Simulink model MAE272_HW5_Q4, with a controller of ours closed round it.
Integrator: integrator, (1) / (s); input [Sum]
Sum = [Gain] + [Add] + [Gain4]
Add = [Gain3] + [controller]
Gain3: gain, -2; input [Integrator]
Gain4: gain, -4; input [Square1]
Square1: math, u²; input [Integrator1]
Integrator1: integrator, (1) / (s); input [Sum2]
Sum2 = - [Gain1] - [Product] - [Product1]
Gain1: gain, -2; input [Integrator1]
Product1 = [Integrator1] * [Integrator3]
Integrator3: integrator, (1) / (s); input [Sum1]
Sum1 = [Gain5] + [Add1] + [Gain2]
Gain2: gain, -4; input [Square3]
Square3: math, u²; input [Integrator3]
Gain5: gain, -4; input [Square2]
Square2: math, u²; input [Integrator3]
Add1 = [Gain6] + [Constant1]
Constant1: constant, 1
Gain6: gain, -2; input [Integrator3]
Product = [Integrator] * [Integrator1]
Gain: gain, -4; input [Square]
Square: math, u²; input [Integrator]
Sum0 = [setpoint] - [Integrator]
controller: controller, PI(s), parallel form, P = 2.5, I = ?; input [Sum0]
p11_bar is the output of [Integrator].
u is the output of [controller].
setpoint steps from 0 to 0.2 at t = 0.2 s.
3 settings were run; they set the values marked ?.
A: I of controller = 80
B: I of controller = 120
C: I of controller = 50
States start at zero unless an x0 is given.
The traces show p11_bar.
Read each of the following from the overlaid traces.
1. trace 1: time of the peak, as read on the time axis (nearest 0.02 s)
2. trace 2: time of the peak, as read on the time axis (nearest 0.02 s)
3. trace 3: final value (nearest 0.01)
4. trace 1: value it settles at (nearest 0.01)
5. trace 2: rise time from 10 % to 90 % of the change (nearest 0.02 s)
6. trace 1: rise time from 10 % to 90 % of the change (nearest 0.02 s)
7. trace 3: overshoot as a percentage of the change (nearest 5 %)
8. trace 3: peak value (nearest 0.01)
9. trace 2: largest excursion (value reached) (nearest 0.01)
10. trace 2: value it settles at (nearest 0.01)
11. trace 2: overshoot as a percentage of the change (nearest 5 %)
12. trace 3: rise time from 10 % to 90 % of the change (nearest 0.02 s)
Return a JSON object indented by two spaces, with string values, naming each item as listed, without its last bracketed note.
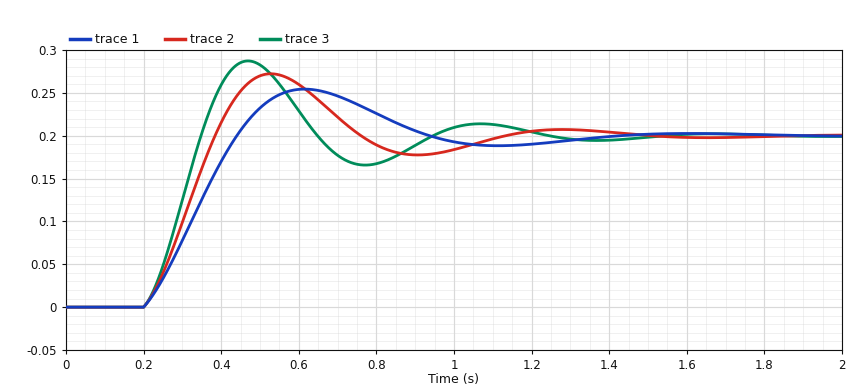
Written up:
{
  "trace 1: time of the peak, as read on the time axis": "0.62 s",
  "trace 2: time of the peak, as read on the time axis": "0.52 s",
  "trace 3: final value": "0.20",
  "trace 1: value it settles at": "0.20",
  "trace 2: rise time from 10 % to 90 % of the change": "0.14 s",
  "trace 1: rise time from 10 % to 90 % of the change": "0.18 s",
  "trace 3: overshoot as a percentage of the change": "45 %",
  "trace 3: peak value": "0.29",
  "trace 2: largest excursion (value reached)": "0.27",
  "trace 2: value it settles at": "0.20",
  "trace 2: overshoot as a percentage of the change": "35 %",
  "trace 3: rise time from 10 % to 90 % of the change": "0.10 s"
}
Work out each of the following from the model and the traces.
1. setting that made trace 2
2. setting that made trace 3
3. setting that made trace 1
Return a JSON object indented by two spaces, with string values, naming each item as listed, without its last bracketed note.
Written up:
{
  "setting that made trace 2": "A",
  "setting that made trace 3": "B",
  "setting that made trace 1": "C"
}
